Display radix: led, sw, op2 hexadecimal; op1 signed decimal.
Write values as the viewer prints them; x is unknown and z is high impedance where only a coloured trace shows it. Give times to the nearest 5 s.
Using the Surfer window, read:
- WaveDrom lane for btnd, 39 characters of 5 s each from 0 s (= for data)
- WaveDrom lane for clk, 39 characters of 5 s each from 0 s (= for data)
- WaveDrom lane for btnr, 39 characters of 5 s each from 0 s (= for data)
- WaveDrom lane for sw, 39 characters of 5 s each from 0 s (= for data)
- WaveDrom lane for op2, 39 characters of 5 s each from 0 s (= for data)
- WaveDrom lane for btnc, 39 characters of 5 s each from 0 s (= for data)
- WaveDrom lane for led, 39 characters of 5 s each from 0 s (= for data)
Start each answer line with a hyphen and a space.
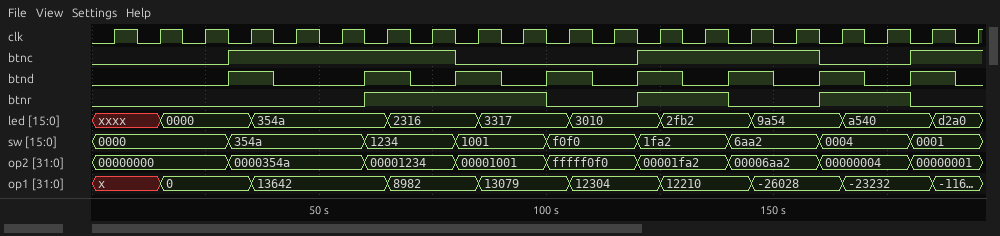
- {name: 'btnd', wave: '0.....1.0...1.0.1.0.1.0.1.0.1.0.1.0.1.0'}
- {name: 'clk', wave: '010101010101010101010101010101010101010'}
- {name: 'btnr', wave: '0...........1.......0...1...0...1...0..'}
- {name: 'sw', wave: '=.....=.....=...=...=...=...=...=...=..', data: '0000 354a 1234 1001 f0f0 1fa2 6aa2 0004 0001'}
- {name: 'op2', wave: '=.....=.....=...=...=...=...=...=...=..', data: '00000000 0000354a 00001234 00001001 fffff0f0 00001fa2 00006aa2 00000004 00000001'}
- {name: 'btnc', wave: '0.....1.........0.......1.......0...1..'}
- {name: 'led', wave: 'x..=...=.....=...=...=...=...=...=...=.', data: '0000 354a 2316 3317 3010 2fb2 9a54 a540 d2a0'}
